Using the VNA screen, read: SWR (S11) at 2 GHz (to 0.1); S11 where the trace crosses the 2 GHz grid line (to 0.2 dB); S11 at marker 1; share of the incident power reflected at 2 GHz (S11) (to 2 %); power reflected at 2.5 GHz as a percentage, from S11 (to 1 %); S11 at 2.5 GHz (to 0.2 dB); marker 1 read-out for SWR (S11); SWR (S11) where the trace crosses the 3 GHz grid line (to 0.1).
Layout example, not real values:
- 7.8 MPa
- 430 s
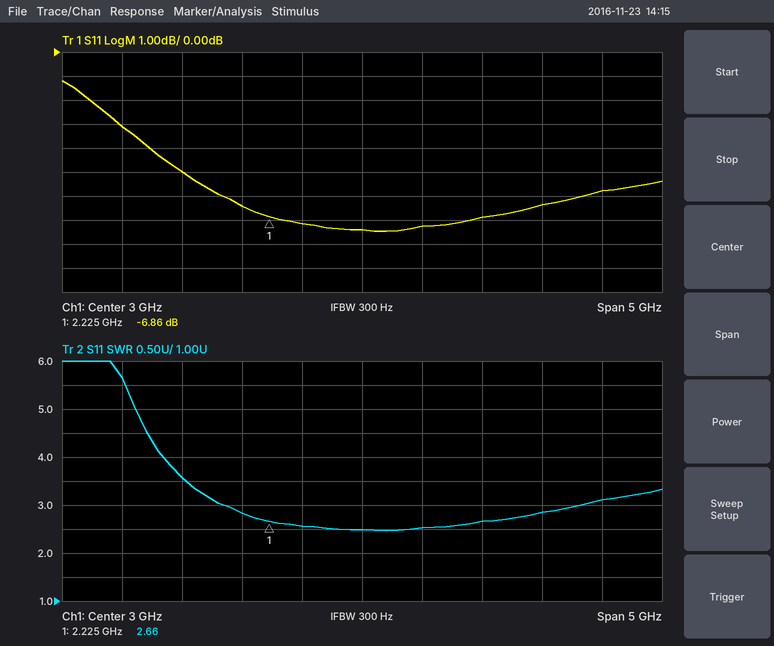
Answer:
- 2.8
- -6.4 dB
- -6.86 dB
- 22 %
- 19 %
- -7.2 dB
- 2.66
- 2.5
